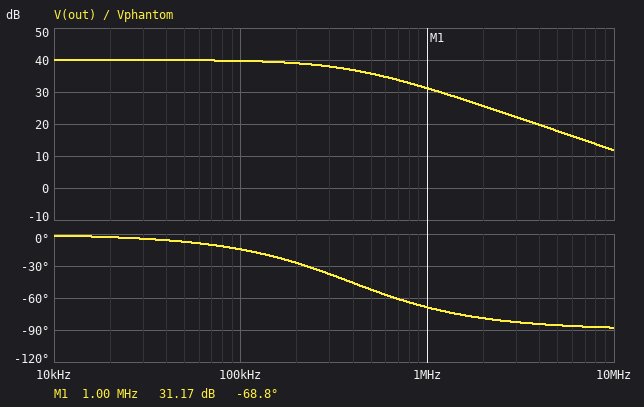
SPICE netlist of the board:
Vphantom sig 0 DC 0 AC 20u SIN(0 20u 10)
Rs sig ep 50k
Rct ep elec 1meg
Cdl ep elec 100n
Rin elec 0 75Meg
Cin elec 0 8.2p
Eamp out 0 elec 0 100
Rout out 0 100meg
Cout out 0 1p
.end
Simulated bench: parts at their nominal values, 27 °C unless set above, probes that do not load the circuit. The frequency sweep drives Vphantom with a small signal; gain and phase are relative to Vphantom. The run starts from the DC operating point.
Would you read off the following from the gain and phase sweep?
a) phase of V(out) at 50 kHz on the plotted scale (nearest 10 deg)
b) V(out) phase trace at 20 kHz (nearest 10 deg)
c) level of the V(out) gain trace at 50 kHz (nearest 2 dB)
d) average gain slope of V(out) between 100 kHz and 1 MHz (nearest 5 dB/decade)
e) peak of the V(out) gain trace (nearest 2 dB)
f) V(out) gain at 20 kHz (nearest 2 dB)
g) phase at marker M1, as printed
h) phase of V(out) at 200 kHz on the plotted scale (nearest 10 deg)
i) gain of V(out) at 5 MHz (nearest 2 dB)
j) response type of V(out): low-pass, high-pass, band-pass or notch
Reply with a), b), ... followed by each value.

a) -10 deg
b) 0 deg
c) 40 dB
d) -10 dB/decade
e) 40 dB
f) 40 dB
g) -68.8 deg
h) -30 deg
i) 18 dB
j) low-pass
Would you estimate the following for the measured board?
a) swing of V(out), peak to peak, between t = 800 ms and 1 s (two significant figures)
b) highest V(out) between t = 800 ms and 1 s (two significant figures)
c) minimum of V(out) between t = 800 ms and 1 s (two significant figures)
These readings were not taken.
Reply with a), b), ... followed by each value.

a) 4.0 mV
b) 2.0 mV
c) -2.0 mV
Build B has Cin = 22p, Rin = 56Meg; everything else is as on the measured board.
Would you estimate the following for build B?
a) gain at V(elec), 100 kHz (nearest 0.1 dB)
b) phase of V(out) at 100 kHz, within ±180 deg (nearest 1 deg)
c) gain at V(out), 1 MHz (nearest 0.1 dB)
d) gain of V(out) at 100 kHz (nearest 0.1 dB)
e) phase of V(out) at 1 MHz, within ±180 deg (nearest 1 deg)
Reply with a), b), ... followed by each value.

a) -1.7 dB
b) -35 deg
c) 23.1 dB
d) 38.3 dB
e) -82 deg
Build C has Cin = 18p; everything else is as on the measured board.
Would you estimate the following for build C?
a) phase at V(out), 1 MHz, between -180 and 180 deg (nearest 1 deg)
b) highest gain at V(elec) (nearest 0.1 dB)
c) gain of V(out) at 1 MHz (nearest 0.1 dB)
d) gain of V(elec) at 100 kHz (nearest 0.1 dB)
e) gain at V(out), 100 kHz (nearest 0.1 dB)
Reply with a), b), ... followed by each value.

a) -80 deg
b) 0 dB
c) 24.8 dB
d) -1.2 dB
e) 38.8 dB
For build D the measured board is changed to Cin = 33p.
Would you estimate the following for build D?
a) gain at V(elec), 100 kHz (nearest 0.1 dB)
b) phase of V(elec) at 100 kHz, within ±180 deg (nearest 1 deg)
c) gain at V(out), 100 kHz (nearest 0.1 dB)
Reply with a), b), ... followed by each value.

a) -3.2 dB
b) -46 deg
c) 36.8 dB
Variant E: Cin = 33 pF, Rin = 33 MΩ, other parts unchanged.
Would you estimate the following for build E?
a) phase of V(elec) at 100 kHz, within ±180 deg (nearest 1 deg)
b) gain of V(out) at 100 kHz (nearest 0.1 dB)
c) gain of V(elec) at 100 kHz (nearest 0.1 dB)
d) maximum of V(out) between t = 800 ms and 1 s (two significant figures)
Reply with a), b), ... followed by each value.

a) -46 deg
b) 36.8 dB
c) -3.2 dB
d) 2.0 mV
